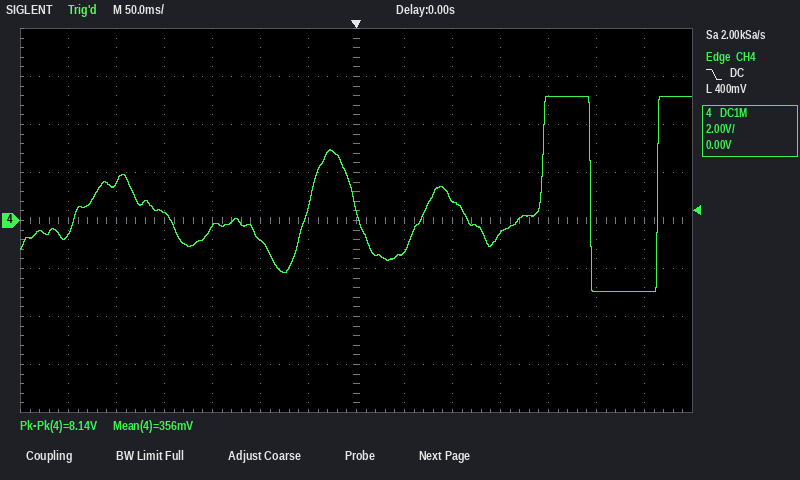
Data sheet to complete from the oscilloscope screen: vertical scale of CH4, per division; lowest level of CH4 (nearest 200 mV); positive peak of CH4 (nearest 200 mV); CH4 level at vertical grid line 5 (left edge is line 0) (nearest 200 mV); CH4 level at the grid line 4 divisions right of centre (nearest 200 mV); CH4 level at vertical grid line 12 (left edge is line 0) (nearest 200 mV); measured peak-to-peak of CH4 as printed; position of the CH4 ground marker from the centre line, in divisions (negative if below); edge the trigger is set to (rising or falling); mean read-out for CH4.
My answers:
2 V
-3.0 V
5.2 V
-800 mV
5.2 V
-3.0 V
8.14 V
0.0 div
falling
356 mV
